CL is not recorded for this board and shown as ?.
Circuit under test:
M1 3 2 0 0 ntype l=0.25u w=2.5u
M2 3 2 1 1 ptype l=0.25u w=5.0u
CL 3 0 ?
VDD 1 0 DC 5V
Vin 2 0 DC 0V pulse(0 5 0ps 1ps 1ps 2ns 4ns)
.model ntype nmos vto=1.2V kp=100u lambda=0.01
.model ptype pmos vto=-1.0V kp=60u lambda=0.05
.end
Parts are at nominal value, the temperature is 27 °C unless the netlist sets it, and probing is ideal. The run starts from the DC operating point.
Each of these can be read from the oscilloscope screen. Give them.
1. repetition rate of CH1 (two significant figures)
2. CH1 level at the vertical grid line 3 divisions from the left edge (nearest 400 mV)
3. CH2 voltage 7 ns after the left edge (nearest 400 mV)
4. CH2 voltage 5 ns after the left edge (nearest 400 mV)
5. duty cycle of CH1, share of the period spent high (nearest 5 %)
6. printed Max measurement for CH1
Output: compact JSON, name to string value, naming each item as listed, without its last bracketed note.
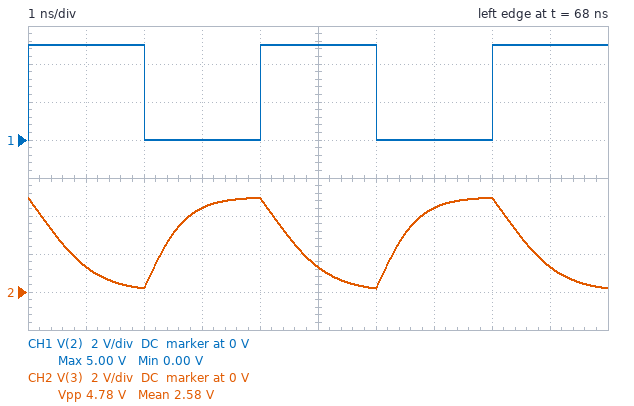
{"repetition rate of CH1": "250 MHz", "CH1 level at the vertical grid line 3 divisions from the left edge": "0 V", "CH2 voltage 7 ns after the left edge": "4.4 V", "CH2 voltage 5 ns after the left edge": "1.2 V", "duty cycle of CH1, share of the period spent high": "50 %", "printed Max measurement for CH1": "5.00 V"}
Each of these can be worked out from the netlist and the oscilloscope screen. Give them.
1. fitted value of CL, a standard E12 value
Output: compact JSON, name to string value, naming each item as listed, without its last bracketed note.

{"fitted value of CL, a standard E12 value": "1.8 pF"}
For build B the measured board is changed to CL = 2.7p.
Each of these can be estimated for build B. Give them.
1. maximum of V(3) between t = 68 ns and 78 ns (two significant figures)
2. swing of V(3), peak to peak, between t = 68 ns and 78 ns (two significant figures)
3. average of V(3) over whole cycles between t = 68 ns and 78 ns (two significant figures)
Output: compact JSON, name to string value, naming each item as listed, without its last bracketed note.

{"maximum of V(3) between t = 68 ns and 78 ns": "4.8 V", "swing of V(3), peak to peak, between t = 68 ns and 78 ns": "4.1 V", "average of V(3) over whole cycles between t = 68 ns and 78 ns": "2.9 V"}
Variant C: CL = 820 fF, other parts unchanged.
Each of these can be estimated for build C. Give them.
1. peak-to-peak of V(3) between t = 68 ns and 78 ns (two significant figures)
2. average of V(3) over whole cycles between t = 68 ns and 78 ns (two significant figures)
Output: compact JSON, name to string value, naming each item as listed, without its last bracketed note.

{"peak-to-peak of V(3) between t = 68 ns and 78 ns": "5.0 V", "average of V(3) over whole cycles between t = 68 ns and 78 ns": "2.6 V"}
